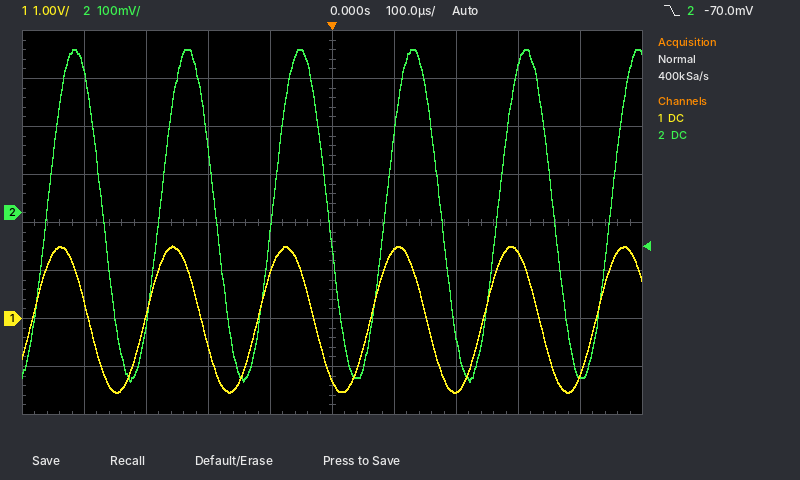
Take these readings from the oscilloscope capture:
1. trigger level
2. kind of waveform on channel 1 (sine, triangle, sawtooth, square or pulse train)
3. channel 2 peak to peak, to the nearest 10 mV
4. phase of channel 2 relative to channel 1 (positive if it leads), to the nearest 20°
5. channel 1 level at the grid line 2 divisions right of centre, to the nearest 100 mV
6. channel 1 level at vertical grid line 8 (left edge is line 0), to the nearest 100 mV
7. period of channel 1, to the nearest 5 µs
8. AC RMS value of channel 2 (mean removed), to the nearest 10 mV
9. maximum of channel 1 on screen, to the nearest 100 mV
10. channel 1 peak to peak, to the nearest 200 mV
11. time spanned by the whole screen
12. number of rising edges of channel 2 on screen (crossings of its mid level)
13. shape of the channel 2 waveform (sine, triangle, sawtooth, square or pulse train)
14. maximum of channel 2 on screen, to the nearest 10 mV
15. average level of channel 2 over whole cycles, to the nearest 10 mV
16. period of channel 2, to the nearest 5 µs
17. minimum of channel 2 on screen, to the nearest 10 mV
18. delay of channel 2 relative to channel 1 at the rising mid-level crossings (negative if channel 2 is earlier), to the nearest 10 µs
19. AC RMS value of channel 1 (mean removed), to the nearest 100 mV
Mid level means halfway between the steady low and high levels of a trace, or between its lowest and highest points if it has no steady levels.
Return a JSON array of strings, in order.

["-70.0 mV", "sine", "690 mV", "-40°", "-1.5 V", "1.4 V", "180 µs", "240 mV", "1.5 V", "3.0 V", "1 ms", "6", "sine", "340 mV", "0 mV", "180 µs", "-350 mV", "+20 µs", "1.1 V"]
